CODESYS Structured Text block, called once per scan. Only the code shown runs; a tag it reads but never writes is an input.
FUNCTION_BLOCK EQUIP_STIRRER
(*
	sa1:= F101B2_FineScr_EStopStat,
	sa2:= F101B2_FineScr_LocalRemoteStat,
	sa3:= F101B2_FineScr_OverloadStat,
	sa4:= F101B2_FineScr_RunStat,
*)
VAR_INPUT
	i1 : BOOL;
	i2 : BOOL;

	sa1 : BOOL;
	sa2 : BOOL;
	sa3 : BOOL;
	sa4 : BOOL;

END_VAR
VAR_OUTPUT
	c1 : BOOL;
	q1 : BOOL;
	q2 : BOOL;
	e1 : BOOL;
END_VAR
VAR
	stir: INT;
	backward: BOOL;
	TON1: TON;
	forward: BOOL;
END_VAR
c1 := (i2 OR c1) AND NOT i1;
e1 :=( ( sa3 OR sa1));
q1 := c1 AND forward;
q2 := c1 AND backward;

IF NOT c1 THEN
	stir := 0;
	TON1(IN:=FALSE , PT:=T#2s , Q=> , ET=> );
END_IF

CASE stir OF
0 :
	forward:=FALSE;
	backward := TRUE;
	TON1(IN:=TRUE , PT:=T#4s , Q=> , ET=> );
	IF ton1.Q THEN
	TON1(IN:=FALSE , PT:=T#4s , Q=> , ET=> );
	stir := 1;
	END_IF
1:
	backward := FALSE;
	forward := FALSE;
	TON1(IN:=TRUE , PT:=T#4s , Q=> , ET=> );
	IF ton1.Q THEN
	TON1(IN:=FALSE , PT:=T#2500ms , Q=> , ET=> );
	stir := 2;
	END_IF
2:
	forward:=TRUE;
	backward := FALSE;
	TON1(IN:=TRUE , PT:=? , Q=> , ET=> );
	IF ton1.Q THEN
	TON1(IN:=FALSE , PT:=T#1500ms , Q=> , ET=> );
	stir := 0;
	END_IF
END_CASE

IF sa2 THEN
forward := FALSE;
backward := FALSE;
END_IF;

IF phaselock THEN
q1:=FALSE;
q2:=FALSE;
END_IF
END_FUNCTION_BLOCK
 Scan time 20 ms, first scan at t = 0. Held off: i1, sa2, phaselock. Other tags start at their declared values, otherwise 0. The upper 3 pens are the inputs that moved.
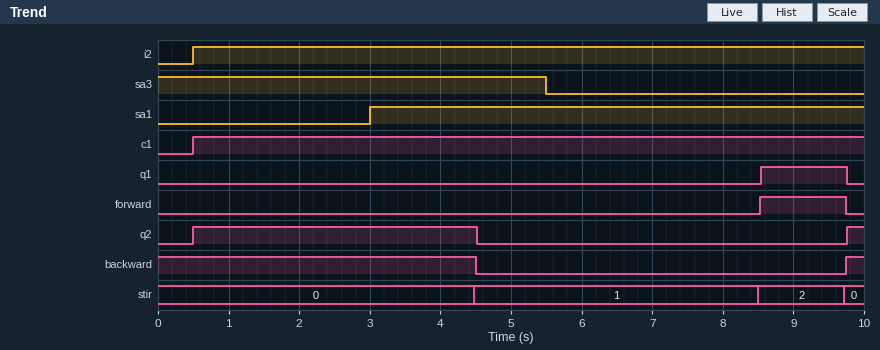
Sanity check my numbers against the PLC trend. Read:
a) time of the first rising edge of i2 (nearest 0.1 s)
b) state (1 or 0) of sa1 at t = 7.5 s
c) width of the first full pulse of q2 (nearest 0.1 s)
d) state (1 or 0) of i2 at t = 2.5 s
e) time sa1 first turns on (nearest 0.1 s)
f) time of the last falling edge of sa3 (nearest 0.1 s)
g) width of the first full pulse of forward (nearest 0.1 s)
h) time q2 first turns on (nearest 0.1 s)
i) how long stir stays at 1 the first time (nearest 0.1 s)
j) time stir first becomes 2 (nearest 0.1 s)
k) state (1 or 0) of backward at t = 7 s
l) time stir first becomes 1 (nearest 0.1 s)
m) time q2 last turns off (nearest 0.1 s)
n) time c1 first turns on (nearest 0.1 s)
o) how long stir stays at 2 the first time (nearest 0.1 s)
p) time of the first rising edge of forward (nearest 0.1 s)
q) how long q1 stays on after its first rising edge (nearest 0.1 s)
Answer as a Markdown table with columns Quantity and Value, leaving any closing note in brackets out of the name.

| Quantity | Value |
|---|---|
| time of the first rising edge of i2 | 0.5 s |
| state (1 or 0) of sa1 at t = 7.5 s | 1 |
| width of the first full pulse of q2 | 4.0 s |
| state (1 or 0) of i2 at t = 2.5 s | 1 |
| time sa1 first turns on | 3.0 s |
| time of the last falling edge of sa3 | 5.5 s |
| width of the first full pulse of forward | 1.2 s |
| time q2 first turns on | 0.5 s |
| how long stir stays at 1 the first time | 4.0 s |
| time stir first becomes 2 | 8.5 s |
| state (1 or 0) of backward at t = 7 s | 0 |
| time stir first becomes 1 | 4.5 s |
| time q2 last turns off | 4.5 s |
| time c1 first turns on | 0.5 s |
| how long stir stays at 2 the first time | 1.2 s |
| time of the first rising edge of forward | 8.5 s |
| how long q1 stays on after its first rising edge | 1.2 s |
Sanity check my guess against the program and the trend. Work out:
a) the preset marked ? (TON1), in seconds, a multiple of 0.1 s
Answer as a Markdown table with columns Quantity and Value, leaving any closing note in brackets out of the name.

| Quantity | Value |
|---|---|
| the preset marked ? (TON1), in seconds, a multiple of 0.1 s | 1.2 s |
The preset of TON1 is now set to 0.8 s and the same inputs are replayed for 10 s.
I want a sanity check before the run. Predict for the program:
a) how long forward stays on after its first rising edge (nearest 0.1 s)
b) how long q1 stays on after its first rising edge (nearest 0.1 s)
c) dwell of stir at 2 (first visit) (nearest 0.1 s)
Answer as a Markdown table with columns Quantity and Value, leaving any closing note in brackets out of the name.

| Quantity | Value |
|---|---|
| how long forward stays on after its first rising edge | 0.8 s |
| how long q1 stays on after its first rising edge | 0.8 s |
| dwell of stir at 2 (first visit) | 0.8 s |
